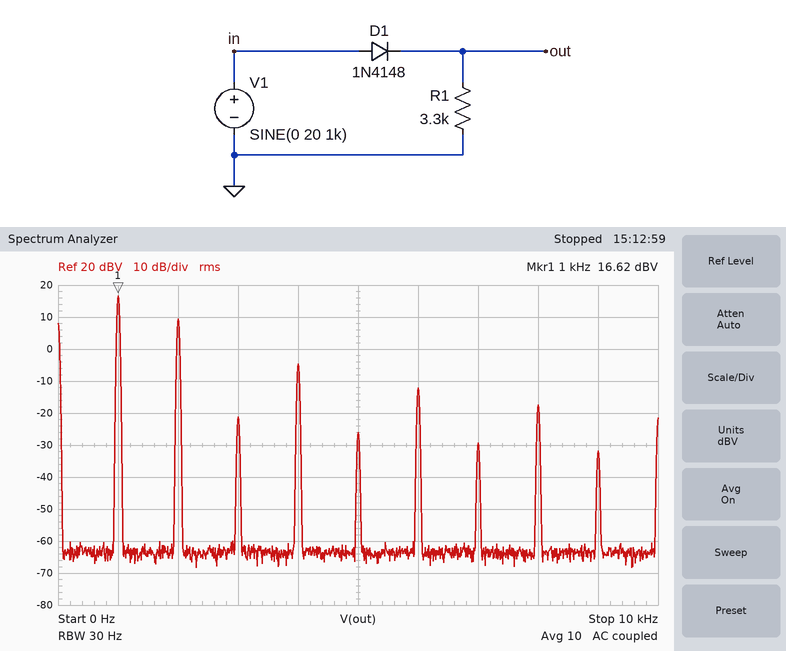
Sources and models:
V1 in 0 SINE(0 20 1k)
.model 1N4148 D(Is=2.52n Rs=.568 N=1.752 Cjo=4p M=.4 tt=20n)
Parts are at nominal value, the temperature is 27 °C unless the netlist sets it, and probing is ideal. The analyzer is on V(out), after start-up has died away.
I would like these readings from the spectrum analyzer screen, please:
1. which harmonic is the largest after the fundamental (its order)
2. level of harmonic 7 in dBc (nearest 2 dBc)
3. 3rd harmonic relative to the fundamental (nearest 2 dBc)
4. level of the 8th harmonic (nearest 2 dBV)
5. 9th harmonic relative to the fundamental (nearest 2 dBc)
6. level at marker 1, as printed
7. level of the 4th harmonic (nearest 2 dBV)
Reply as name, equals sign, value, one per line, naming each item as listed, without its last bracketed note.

which harmonic is the largest after the fundamental = 2
level of harmonic 7 in dBc = -46 dBc
3rd harmonic relative to the fundamental = -38 dBc
level of the 8th harmonic = -18 dBV
9th harmonic relative to the fundamental = -48 dBc
level at marker 1, as printed = 16.62 dBV
level of the 4th harmonic = -4 dBV
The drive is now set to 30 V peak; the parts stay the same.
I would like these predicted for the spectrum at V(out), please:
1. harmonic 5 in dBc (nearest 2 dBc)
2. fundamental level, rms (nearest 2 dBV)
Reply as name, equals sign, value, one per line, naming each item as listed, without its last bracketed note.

harmonic 5 in dBc = -46 dBc
fundamental level, rms = 20 dBV
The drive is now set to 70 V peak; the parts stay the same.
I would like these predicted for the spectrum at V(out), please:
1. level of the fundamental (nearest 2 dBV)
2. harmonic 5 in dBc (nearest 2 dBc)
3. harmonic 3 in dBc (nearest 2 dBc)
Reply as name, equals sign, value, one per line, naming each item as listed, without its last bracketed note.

level of the fundamental = 28 dBV
harmonic 5 in dBc = -52 dBc
harmonic 3 in dBc = -48 dBc
